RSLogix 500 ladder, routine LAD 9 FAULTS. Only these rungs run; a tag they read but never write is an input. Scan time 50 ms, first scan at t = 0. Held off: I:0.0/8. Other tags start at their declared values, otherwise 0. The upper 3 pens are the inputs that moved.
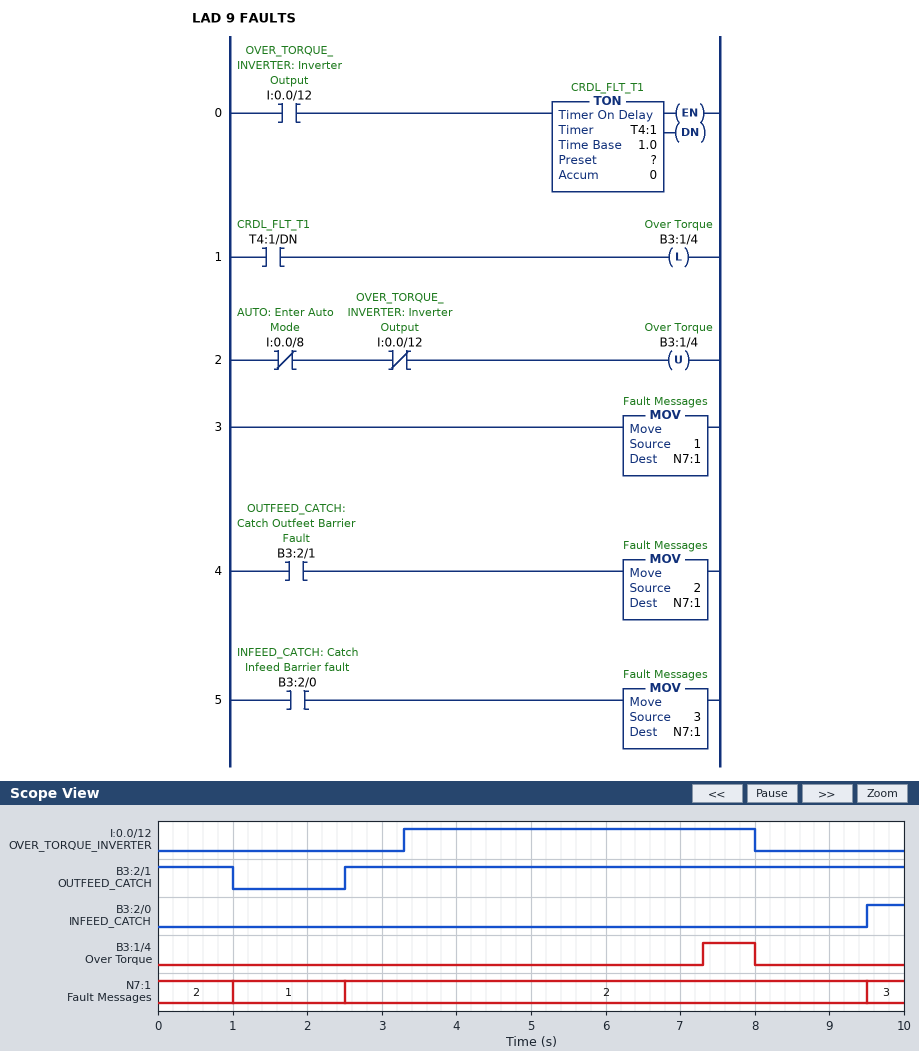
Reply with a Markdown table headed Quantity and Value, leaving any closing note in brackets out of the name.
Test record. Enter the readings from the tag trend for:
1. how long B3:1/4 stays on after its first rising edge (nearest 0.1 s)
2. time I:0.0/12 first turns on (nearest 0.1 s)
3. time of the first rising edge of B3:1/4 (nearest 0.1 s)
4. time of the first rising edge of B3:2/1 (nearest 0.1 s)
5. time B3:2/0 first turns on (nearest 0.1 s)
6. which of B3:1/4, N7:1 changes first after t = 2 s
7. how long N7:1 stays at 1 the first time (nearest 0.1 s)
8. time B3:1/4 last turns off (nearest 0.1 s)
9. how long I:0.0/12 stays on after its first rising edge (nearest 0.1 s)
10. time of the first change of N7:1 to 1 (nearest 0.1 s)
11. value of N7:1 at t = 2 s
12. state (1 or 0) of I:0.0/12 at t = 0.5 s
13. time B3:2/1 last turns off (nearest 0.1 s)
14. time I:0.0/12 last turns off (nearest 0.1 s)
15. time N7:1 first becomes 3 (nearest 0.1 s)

| Quantity | Value |
|---|---|
| how long B3:1/4 stays on after its first rising edge | 0.7 s |
| time I:0.0/12 first turns on | 3.3 s |
| time of the first rising edge of B3:1/4 | 7.3 s |
| time of the first rising edge of B3:2/1 | 2.5 s |
| time B3:2/0 first turns on | 9.5 s |
| which of B3:1/4, N7:1 changes first after t = 2 s | N7:1 |
| how long N7:1 stays at 1 the first time | 1.5 s |
| time B3:1/4 last turns off | 8.0 s |
| how long I:0.0/12 stays on after its first rising edge | 4.7 s |
| time of the first change of N7:1 to 1 | 1.0 s |
| value of N7:1 at t = 2 s | 1 |
| state (1 or 0) of I:0.0/12 at t = 0.5 s | 0 |
| time B3:2/1 last turns off | 1.0 s |
| time I:0.0/12 last turns off | 8.0 s |
| time N7:1 first becomes 3 | 9.5 s |
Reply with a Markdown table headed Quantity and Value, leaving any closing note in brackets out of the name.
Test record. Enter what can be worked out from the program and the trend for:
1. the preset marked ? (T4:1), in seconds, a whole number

| Quantity | Value |
|---|---|
| the preset marked ? (T4:1), in seconds, a whole number | 4 s |
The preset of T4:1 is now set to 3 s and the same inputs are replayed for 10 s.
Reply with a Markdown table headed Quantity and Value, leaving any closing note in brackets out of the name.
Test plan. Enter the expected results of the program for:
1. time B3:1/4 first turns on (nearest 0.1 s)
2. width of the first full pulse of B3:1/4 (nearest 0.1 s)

| Quantity | Value |
|---|---|
| time B3:1/4 first turns on | 6.3 s |
| width of the first full pulse of B3:1/4 | 1.7 s |
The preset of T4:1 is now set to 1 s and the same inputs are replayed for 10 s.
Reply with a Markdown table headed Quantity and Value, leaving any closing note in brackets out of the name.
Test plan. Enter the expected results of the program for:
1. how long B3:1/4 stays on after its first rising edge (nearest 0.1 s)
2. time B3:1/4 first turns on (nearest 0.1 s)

| Quantity | Value |
|---|---|
| how long B3:1/4 stays on after its first rising edge | 3.7 s |
| time B3:1/4 first turns on | 4.3 s |
